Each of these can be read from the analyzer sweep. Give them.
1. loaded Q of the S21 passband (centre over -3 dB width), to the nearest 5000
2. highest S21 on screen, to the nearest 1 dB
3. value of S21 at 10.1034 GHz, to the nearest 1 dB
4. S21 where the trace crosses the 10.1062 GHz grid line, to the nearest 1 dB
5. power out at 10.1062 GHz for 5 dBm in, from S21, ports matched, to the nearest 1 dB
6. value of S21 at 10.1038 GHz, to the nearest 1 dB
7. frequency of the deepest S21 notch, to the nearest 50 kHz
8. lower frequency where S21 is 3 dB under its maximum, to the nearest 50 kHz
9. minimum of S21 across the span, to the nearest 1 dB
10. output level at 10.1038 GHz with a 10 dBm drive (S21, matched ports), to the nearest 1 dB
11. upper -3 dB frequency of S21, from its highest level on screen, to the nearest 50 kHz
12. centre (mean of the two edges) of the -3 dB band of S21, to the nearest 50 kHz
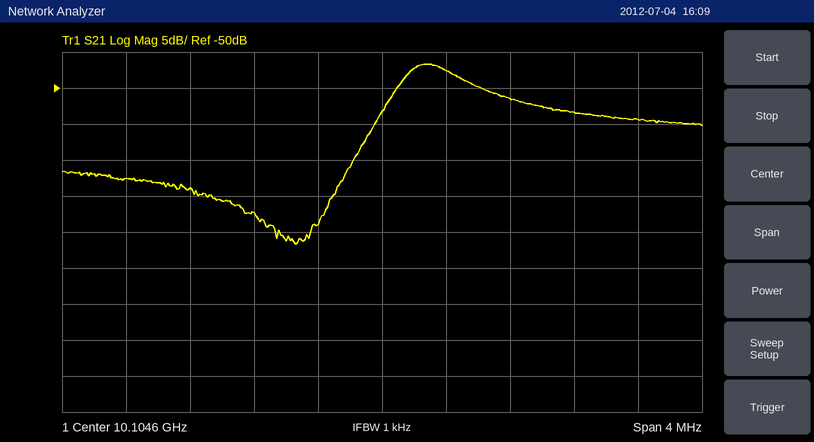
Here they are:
20000
-47 dB
-64 dB
-54 dB
-49 dBm
-67 dB
10.10405 GHz
10.10470 GHz
-72 dB
-57 dBm
10.10520 GHz
10.10495 GHz
